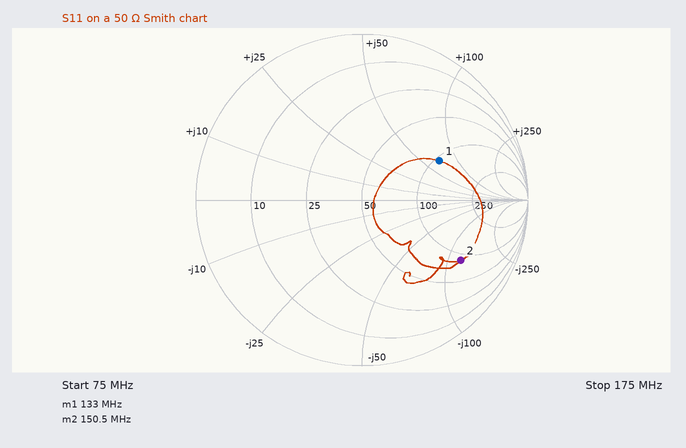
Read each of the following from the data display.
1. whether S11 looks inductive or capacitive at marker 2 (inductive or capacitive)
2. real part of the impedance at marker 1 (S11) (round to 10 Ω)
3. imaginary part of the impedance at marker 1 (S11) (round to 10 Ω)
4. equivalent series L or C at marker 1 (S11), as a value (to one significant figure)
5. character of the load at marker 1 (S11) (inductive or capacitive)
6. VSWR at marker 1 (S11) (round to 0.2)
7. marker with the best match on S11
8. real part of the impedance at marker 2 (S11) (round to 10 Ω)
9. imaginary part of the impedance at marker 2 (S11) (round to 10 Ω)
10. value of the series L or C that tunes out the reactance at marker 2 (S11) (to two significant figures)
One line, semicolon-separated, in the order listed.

capacitive; 110 Ω; +70 Ω; 80 nH; inductive; 3.2; marker 1; 90 Ω; -120 Ω; 130 nH
